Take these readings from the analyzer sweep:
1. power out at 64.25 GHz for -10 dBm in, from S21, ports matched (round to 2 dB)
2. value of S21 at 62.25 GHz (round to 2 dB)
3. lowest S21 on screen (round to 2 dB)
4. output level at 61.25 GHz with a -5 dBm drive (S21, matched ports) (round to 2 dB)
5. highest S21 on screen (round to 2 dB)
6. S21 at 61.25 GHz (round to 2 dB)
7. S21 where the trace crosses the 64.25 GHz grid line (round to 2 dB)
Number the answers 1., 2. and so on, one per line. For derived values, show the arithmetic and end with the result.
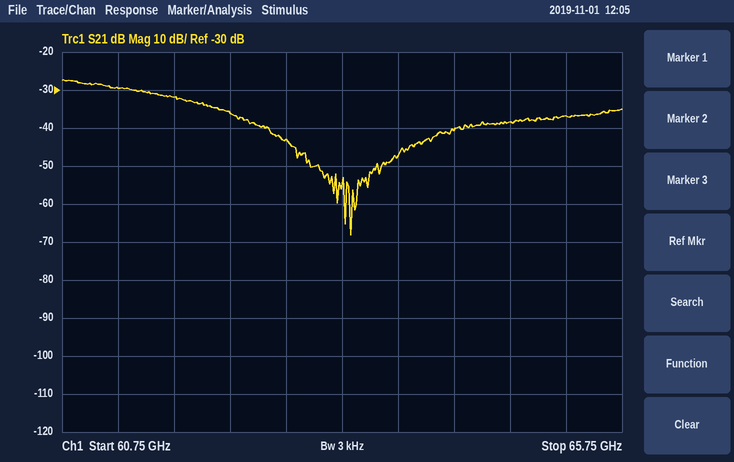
1. -10 dBm + (-40 dB) = -50 dBm
2. -36 dB
3. -68 dB
4. -5 dBm + (-30 dB) = -34 dBm
5. -28 dB
6. -30 dB
7. -40 dB
